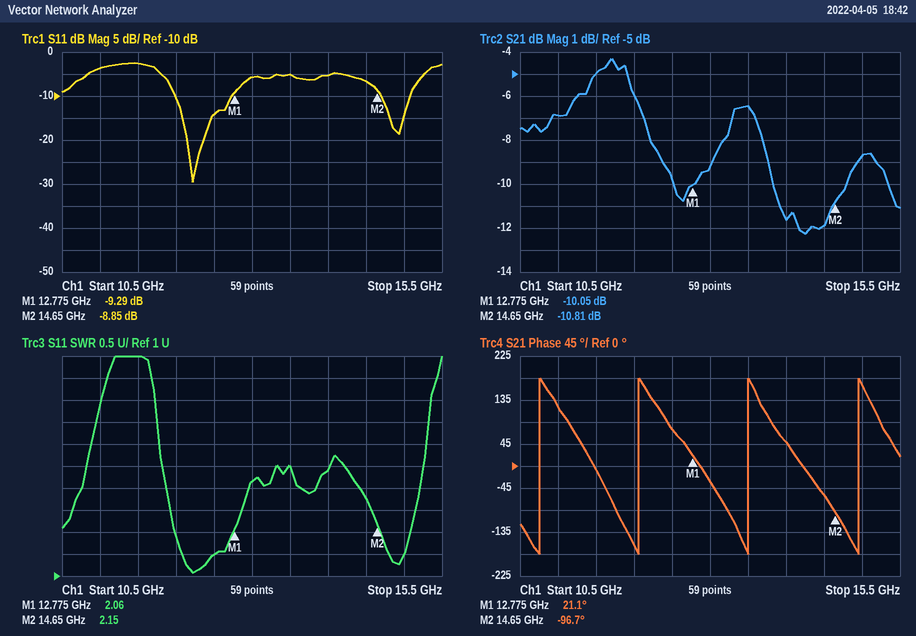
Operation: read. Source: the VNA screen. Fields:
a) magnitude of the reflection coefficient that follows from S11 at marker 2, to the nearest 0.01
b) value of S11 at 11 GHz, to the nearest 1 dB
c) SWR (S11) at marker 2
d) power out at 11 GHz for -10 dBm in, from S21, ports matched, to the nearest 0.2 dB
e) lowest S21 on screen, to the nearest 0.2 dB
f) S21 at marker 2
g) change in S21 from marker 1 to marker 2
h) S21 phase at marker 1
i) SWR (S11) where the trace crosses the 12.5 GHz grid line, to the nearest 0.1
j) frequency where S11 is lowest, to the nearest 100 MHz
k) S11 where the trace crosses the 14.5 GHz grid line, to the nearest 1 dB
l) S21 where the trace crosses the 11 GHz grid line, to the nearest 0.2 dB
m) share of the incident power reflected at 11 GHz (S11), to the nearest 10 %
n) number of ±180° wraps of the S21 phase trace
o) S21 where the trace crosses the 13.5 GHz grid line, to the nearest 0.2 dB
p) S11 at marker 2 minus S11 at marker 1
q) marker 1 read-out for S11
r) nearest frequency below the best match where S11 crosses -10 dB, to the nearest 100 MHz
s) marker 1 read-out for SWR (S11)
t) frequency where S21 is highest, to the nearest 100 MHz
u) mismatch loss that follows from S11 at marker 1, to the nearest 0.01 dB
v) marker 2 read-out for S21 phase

0.36
-4 dB
2.15
-16.8 dBm
-12.2 dB
-10.81 dB
-0.76 dB
21.1°
1.5
12.2 GHz
-7 dB
-6.8 dB
40 %
4
-6.4 dB
0.44 dB
-9.29 dB
12.0 GHz
2.06
11.7 GHz
0.54 dB
-96.7°
